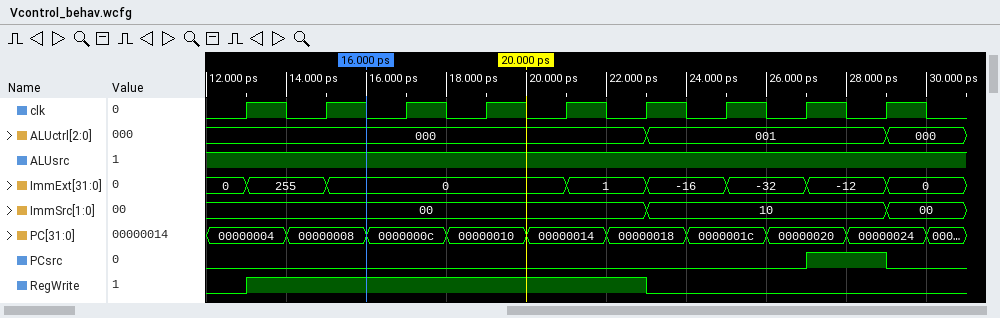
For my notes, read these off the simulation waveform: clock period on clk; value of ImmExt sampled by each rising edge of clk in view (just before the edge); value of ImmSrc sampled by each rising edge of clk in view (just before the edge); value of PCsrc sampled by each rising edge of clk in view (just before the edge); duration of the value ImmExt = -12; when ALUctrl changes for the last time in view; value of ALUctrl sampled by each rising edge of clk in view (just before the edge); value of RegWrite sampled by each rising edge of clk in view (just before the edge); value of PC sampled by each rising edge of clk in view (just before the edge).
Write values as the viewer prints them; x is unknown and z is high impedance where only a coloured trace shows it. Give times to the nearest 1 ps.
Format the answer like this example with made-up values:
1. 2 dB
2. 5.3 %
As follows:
1. 2 ps
2. 0, 255, 0, 0, 0, 1, -16, -32, -12
3. 00, 00, 00, 00, 00, 00, 10, 10, 10
4. 0 0 0 0 0 0 0 0 1
5. 2 ps
6. 29 ps
7. 000, 000, 000, 000, 000, 000, 001, 001, 001
8. 0 1 1 1 1 1 0 0 0
9. 00000004, 00000008, 0000000c, 00000010, 00000014, 00000018, 0000001c, 00000020, 00000024
